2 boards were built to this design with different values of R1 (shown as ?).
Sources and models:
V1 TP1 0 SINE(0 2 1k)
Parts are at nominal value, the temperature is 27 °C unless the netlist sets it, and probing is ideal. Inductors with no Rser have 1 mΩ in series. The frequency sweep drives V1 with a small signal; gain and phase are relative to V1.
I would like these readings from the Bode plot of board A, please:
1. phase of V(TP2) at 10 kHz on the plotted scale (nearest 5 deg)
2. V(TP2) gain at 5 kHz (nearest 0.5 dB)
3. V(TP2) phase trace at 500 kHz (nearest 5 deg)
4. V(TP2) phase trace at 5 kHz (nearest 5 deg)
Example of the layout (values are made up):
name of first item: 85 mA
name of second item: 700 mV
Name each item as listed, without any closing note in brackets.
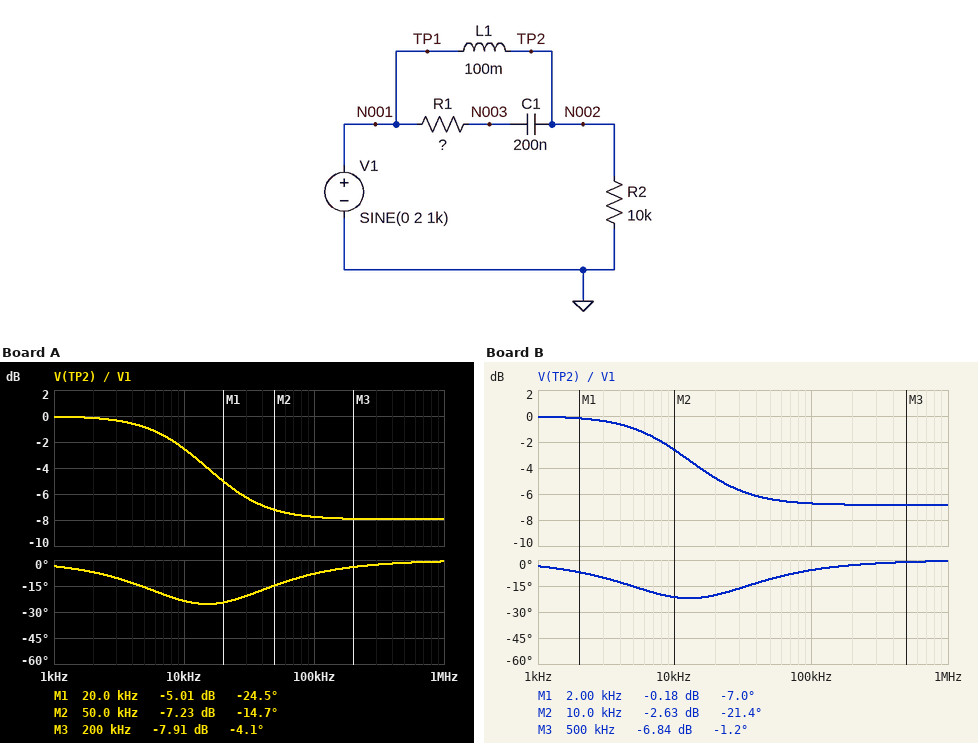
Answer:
phase of V(TP2) at 10 kHz on the plotted scale: -25 deg
V(TP2) gain at 5 kHz: -1.0 dB
V(TP2) phase trace at 500 kHz: 0 deg
V(TP2) phase trace at 5 kHz: -15 deg
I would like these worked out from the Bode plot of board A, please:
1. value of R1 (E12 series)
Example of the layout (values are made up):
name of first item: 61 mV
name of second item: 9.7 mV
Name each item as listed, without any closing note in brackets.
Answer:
value of R1: 15 kΩ
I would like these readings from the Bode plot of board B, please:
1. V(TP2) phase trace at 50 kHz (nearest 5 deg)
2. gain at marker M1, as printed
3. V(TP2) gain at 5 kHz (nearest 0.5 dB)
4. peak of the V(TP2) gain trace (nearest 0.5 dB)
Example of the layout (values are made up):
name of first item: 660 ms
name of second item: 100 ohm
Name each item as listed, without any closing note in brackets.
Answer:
V(TP2) phase trace at 50 kHz: -10 deg
gain at marker M1, as printed: -0.18 dB
V(TP2) gain at 5 kHz: -1.0 dB
peak of the V(TP2) gain trace: 0 dB
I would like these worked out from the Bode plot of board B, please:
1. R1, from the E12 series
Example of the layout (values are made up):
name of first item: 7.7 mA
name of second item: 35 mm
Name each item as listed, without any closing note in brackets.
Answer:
R1, from the E12 series: 12 kΩ
